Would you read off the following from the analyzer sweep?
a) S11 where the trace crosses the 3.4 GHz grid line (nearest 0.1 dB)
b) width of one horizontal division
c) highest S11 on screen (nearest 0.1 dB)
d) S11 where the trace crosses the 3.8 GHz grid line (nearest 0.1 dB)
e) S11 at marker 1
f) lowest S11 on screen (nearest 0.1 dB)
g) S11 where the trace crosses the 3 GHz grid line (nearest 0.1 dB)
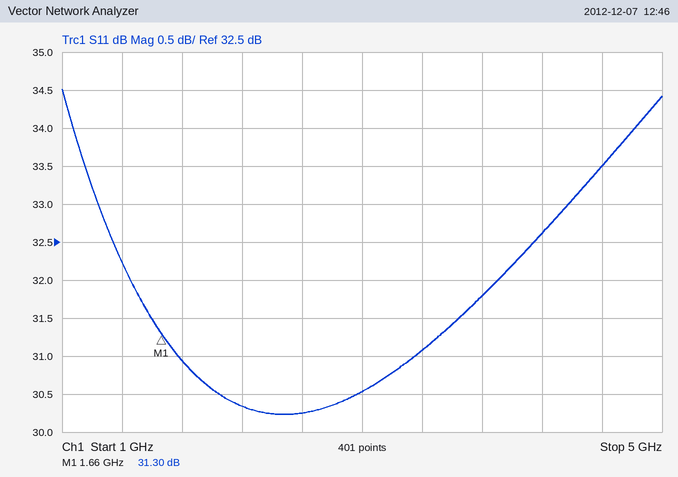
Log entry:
31.1 dB
400 MHz
34.5 dB
31.8 dB
31.30 dB
30.2 dB
30.5 dB
